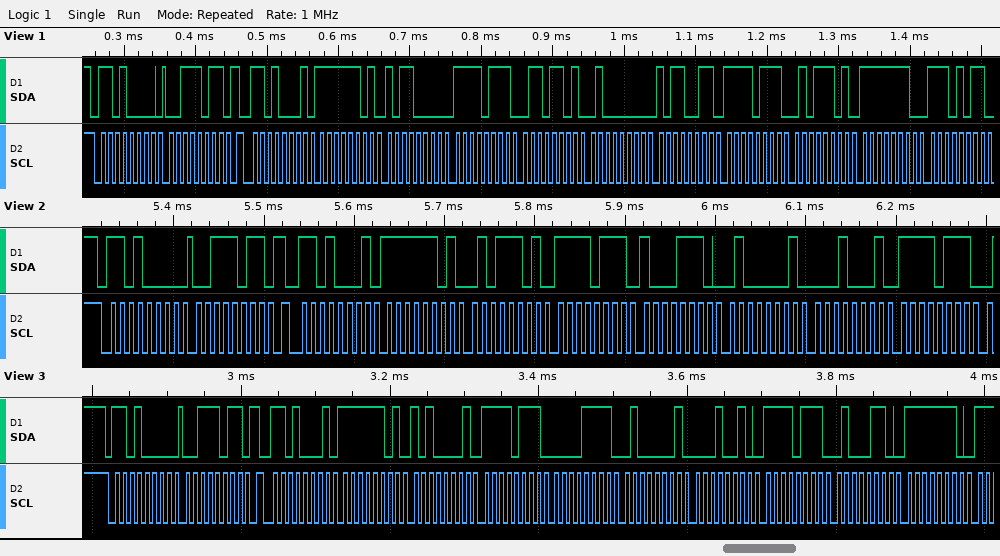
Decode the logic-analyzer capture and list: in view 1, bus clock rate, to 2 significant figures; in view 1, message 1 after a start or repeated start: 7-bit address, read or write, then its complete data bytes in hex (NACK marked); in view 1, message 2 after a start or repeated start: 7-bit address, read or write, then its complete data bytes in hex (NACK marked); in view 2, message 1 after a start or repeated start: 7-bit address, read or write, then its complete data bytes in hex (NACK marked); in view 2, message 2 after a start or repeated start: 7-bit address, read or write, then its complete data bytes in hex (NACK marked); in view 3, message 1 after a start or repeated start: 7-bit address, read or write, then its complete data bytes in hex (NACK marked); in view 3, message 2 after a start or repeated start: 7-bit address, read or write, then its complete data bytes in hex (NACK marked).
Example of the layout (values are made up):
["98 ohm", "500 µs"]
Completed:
["100 kHz", "0x68 write: 3B", "0x68 read: FD B0 F7 6D 40 B3 F7 5D FE EB", "0x68 write: 3B", "0x68 read: FD 5D F7 8E 41 11 F7", "0x68 write: 3B", "0x68 read: FD A1 F7 0F 41 12 F7 46 FE"]
